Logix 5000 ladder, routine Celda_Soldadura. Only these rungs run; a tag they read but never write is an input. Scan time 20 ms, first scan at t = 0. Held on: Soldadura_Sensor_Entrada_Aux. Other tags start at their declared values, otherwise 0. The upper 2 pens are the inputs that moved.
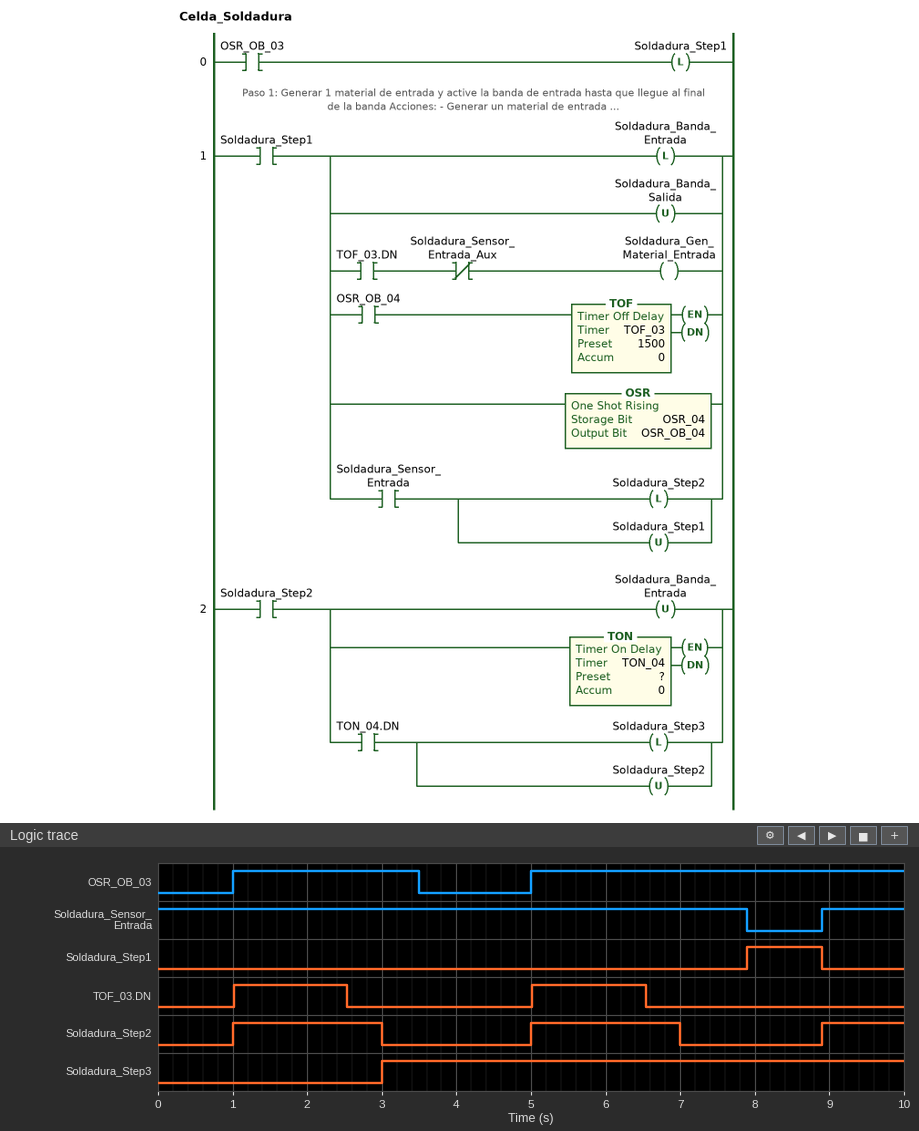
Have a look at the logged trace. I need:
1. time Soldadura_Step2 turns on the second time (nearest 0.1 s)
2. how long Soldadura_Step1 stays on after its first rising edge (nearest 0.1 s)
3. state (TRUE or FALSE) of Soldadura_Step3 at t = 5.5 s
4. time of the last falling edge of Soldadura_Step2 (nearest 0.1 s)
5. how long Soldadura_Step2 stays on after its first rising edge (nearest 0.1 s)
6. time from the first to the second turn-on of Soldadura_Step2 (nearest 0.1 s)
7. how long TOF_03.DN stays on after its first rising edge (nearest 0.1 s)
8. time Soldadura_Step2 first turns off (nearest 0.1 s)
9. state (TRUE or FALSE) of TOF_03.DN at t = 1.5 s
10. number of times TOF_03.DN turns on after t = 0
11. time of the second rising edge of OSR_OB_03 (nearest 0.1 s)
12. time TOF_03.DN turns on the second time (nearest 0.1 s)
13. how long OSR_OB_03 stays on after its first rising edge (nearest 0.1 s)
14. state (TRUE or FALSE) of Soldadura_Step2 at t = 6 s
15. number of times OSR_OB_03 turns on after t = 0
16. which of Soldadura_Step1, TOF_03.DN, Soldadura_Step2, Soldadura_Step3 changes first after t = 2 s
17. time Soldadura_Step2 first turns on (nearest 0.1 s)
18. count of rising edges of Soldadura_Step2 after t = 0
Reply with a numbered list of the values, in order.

1. 5.0 s
2. 1.0 s
3. TRUE
4. 7.0 s
5. 2.0 s
6. 4.0 s
7. 1.5 s
8. 3.0 s
9. TRUE
10. 2
11. 5.0 s
12. 5.0 s
13. 2.5 s
14. TRUE
15. 2
16. TOF_03.DN
17. 1.0 s
18. 3
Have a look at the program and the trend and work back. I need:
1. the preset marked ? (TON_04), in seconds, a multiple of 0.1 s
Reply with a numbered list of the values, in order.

1. 2.0 s
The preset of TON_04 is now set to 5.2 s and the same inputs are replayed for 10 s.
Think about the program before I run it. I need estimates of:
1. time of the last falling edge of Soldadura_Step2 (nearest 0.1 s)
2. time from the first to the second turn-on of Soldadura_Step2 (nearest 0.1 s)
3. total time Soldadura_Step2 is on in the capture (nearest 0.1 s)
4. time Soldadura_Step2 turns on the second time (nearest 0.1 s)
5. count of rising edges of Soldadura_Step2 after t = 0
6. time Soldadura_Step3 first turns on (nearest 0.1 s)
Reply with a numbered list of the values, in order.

1. 6.2 s
2. 7.9 s
3. 6.3 s
4. 8.9 s
5. 2
6. 6.2 s
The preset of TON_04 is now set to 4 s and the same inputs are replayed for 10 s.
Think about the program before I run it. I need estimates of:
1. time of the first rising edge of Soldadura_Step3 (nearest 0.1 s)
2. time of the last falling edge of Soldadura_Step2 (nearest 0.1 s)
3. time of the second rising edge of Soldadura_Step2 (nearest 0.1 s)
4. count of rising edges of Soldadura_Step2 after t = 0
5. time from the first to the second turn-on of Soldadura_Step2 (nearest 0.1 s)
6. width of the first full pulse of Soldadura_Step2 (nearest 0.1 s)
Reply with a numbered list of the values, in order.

1. 5.0 s
2. 5.0 s
3. 8.9 s
4. 2
5. 7.9 s
6. 4.0 s
